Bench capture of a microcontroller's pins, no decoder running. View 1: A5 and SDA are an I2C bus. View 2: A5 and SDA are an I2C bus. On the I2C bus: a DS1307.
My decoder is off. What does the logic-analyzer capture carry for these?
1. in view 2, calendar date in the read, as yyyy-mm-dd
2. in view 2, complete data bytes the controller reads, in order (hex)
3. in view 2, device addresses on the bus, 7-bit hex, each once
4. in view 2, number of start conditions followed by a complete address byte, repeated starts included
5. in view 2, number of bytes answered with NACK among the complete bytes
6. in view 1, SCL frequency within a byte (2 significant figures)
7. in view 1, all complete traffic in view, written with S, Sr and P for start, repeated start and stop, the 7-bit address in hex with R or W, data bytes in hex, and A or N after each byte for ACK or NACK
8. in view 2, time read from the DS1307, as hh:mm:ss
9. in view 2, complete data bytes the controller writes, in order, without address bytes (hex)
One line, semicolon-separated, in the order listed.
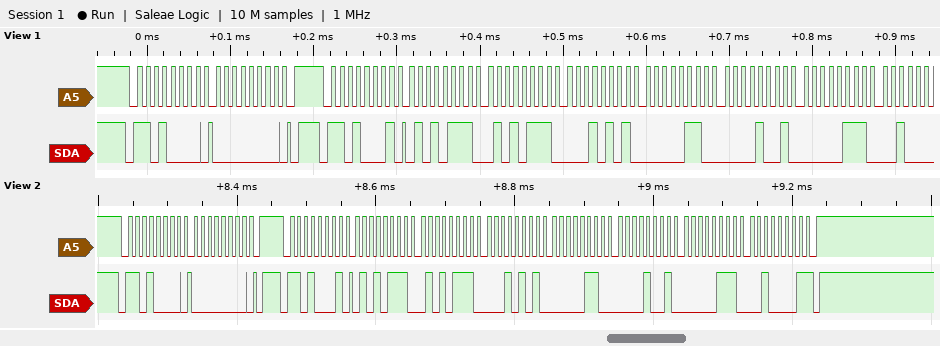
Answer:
2021-07-09; 57 57 15 06 09 07 21; 0x68; 2; 1; 100 kHz; S 68W A 00 A P S 68R A 57 A 57 A 15 A 06 A 09 A 07 A; 15:57:57; 00
